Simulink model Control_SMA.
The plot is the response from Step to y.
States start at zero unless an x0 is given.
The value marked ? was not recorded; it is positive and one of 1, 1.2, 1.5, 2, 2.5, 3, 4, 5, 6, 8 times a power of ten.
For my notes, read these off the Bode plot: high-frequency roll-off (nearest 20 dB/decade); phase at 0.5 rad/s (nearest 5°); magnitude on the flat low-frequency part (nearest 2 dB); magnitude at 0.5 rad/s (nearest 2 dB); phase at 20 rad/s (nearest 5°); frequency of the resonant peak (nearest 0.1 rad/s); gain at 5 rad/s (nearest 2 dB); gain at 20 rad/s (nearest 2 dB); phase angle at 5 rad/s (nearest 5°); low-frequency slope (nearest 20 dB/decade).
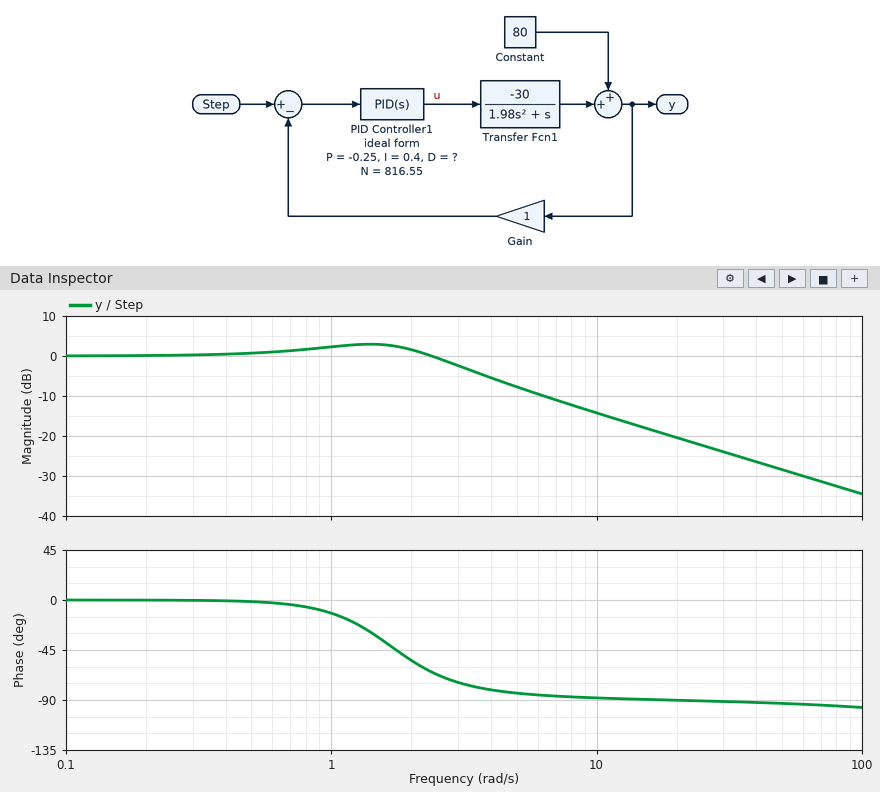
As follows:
-20 dB/decade
0°
0 dB
0 dB
-90°
1.4 rad/s
-8 dB
-20 dB
-85°
0 dB/decade
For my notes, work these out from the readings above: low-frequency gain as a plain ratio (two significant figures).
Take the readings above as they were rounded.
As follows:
1.0
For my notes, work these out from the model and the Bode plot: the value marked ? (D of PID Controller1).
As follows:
0.5
